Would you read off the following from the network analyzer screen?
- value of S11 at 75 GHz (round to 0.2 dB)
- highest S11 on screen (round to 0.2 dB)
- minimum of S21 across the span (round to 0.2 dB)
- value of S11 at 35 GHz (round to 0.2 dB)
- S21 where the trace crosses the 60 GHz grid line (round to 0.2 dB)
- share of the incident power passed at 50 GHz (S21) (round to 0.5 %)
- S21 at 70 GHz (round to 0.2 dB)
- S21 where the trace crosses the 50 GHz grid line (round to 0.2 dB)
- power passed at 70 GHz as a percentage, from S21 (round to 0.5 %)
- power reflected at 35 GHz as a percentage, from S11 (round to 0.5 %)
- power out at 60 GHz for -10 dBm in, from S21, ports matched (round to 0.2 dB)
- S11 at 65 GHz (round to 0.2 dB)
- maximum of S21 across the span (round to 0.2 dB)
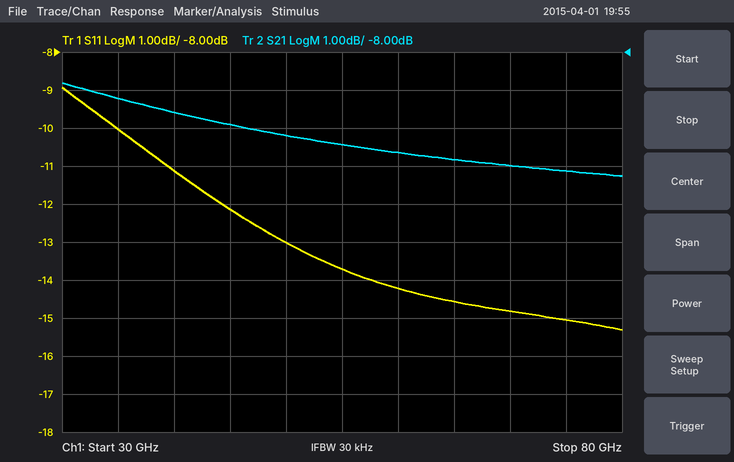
-15.0 dB
-9.0 dB
-11.2 dB
-10.0 dB
-10.6 dB
9.5 %
-11.0 dB
-10.2 dB
8.0 %
10.0 %
-20.6 dBm
-14.6 dB
-8.8 dB
